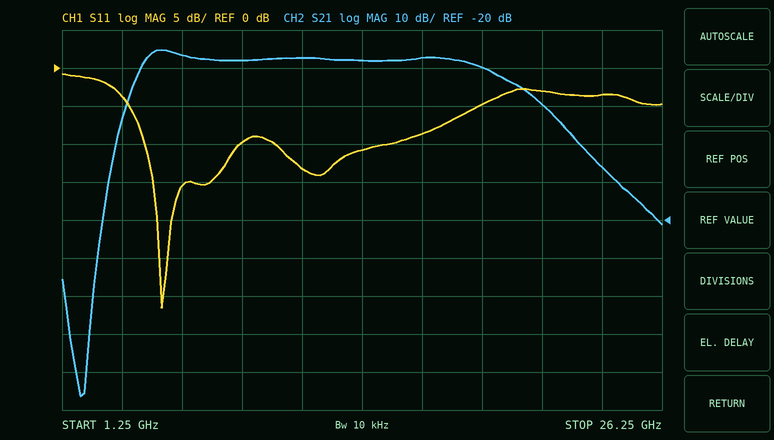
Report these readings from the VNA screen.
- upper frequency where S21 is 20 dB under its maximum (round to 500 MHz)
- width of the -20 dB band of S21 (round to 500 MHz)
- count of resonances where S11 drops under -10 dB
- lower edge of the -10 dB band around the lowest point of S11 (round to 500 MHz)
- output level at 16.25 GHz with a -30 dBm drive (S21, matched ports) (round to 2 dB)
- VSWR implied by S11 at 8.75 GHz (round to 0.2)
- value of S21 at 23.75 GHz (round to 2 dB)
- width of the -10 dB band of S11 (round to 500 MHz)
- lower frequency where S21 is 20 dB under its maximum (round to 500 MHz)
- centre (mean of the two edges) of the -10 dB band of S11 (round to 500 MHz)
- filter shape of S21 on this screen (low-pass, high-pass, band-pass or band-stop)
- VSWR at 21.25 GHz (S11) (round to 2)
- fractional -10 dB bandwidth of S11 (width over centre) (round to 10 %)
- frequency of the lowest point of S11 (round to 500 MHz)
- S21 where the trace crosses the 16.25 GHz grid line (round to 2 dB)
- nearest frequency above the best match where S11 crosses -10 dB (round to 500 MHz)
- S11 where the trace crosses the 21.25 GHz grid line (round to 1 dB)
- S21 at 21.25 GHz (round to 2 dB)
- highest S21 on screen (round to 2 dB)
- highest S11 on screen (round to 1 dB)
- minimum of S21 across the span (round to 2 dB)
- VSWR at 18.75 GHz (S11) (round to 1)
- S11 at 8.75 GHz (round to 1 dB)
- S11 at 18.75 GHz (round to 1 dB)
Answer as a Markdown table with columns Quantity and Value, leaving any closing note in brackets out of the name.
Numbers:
| Quantity | Value |
|---|---|
| upper frequency where S21 is 20 dB under its maximum | 22.0 GHz |
| width of the -20 dB band of S21 | 18.5 GHz |
| count of resonances where S11 drops under -10 dB | 2 |
| lower edge of the -10 dB band around the lowest point of S11 | 4.5 GHz |
| output level at 16.25 GHz with a -30 dBm drive (S21, matched ports) | -8 dBm |
| VSWR implied by S11 at 8.75 GHz | 2.0 |
| value of S21 at 23.75 GHz | -6 dB |
| width of the -10 dB band of S11 | 4.0 GHz |
| lower frequency where S21 is 20 dB under its maximum | 3.5 GHz |
| centre (mean of the two edges) of the -10 dB band of S11 | 6.5 GHz |
| filter shape of S21 on this screen | band-pass |
| VSWR at 21.25 GHz (S11) | 6 |
| fractional -10 dB bandwidth of S11 (width over centre) | 60 % |
| frequency of the lowest point of S11 | 5.5 GHz |
| S21 where the trace crosses the 16.25 GHz grid line | 22 dB |
| nearest frequency above the best match where S11 crosses -10 dB | 8.5 GHz |
| S11 where the trace crosses the 21.25 GHz grid line | -3 dB |
| S21 at 21.25 GHz | 10 dB |
| highest S21 on screen | 24 dB |
| highest S11 on screen | -1 dB |
| minimum of S21 across the span | -66 dB |
| VSWR at 18.75 GHz (S11) | 4 |
| S11 at 8.75 GHz | -10 dB |
| S11 at 18.75 GHz | -5 dB |
